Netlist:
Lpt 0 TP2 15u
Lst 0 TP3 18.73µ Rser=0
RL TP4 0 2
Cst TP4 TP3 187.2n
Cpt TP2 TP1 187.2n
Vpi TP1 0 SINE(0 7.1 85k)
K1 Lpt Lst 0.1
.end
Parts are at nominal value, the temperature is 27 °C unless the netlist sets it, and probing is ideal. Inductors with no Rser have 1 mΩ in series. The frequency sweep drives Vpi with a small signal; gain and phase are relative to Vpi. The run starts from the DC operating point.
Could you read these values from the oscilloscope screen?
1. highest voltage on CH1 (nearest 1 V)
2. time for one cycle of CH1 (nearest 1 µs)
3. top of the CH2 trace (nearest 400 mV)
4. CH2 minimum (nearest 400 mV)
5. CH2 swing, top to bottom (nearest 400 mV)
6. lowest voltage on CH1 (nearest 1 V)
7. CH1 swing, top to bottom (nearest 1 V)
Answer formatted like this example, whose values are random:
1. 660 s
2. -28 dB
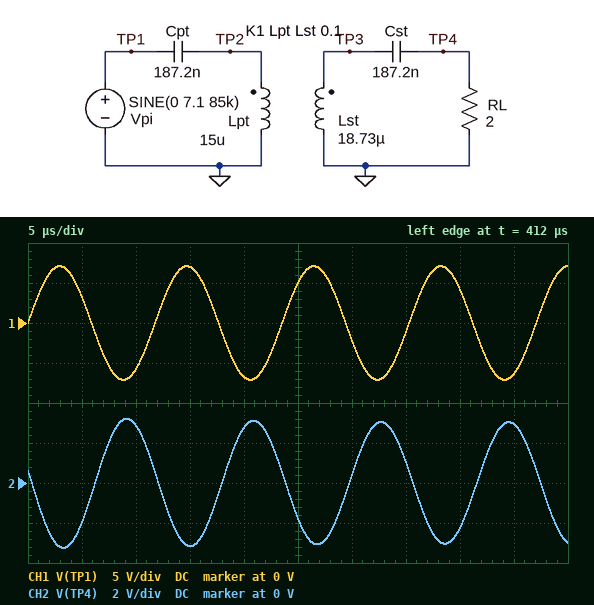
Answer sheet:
1. 7 V
2. 12 µs
3. 3.2 V
4. -3.2 V
5. 6.4 V
6. -7 V
7. 14 V
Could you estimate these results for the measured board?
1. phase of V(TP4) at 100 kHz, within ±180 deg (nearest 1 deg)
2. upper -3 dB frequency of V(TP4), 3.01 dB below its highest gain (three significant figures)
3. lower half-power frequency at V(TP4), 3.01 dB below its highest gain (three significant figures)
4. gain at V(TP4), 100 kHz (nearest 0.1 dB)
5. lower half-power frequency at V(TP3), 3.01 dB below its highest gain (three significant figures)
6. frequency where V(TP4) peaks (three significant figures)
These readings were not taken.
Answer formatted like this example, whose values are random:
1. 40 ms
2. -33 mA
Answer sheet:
1. -46 deg
2. 97.4 kHz
3. 95.2 kHz
4. -2.0 dB
5. 95.2 kHz
6. 96.4 kHz
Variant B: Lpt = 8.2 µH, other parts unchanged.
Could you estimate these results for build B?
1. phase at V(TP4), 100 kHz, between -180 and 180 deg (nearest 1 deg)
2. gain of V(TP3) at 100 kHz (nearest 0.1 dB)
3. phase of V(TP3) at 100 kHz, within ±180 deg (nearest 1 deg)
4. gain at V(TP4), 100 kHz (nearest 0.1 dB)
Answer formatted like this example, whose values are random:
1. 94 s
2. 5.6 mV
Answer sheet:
1. 120 deg
2. -5.9 dB
3. 43 deg
4. -18.7 dB
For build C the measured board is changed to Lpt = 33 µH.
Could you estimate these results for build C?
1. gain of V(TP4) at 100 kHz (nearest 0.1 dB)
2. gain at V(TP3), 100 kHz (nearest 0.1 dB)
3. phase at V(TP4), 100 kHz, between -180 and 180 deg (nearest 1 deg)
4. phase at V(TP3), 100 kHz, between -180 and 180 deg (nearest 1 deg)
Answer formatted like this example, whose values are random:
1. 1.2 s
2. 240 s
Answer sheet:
1. -23.1 dB
2. -10.3 dB
3. -57 deg
4. -134 deg
